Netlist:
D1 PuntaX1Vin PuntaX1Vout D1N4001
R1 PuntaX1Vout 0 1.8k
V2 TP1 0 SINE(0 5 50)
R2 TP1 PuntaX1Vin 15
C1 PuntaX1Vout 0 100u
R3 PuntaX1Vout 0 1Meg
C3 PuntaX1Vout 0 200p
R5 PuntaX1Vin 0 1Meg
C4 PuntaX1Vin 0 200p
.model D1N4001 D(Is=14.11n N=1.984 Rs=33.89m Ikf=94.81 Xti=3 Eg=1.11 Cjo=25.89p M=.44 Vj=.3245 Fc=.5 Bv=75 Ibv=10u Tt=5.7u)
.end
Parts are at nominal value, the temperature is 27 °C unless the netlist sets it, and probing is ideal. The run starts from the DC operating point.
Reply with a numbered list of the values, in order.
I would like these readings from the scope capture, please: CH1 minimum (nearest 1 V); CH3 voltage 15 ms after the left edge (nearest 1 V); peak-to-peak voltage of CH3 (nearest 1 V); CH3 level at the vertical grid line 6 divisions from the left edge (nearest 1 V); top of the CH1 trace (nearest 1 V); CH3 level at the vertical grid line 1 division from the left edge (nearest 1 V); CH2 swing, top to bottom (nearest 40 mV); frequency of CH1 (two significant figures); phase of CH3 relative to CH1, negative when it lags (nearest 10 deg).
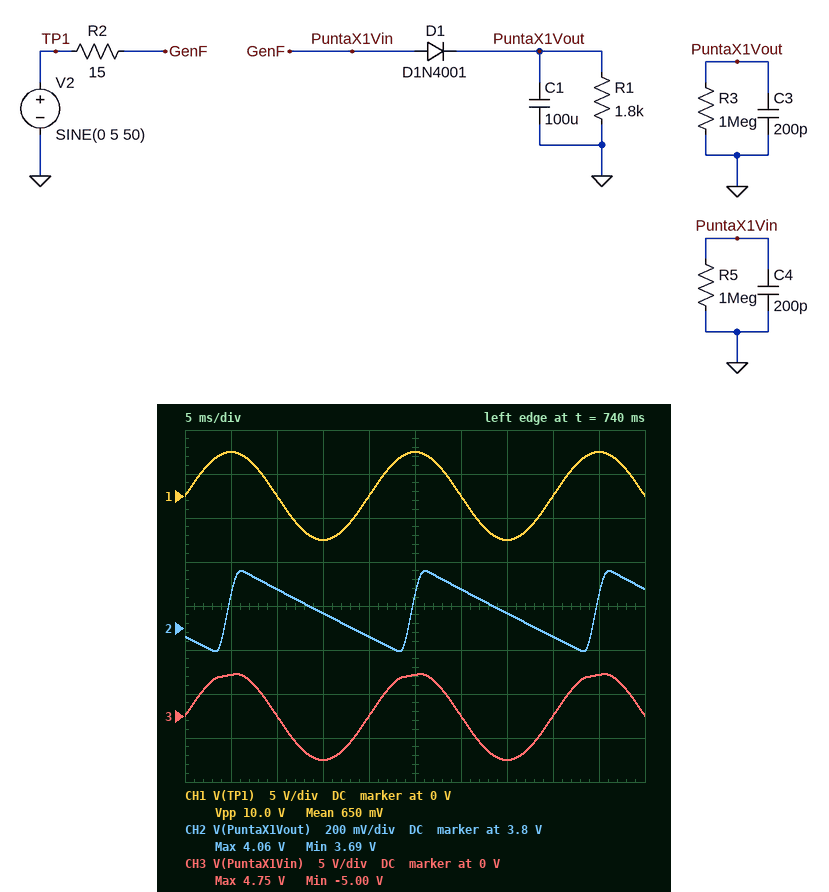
1. -5 V
2. -5 V
3. 10 V
4. 0 V
5. 5 V
6. 5 V
7. 360 mV
8. 50 Hz
9. 0 deg
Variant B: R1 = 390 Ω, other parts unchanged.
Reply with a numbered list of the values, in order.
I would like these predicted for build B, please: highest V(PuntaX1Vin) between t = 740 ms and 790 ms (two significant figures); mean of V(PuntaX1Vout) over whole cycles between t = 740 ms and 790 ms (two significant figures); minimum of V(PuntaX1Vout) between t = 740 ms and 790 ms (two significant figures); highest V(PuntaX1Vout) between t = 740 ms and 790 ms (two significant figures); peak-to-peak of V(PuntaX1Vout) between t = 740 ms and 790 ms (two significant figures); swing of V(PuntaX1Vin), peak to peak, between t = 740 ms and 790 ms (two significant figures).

1. 4.5 V
2. 3.1 V
3. 2.5 V
4. 3.8 V
5. 1.3 V
6. 9.5 V
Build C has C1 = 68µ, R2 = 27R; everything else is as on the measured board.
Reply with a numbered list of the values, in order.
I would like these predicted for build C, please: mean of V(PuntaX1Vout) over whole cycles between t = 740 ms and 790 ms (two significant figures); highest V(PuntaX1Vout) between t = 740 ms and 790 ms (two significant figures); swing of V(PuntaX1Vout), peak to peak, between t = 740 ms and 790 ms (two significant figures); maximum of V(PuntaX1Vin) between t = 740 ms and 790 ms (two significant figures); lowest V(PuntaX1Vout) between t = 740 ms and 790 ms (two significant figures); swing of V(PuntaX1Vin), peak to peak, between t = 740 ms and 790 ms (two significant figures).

1. 3.7 V
2. 4.0 V
3. 500 mV
4. 4.6 V
5. 3.5 V
6. 9.6 V
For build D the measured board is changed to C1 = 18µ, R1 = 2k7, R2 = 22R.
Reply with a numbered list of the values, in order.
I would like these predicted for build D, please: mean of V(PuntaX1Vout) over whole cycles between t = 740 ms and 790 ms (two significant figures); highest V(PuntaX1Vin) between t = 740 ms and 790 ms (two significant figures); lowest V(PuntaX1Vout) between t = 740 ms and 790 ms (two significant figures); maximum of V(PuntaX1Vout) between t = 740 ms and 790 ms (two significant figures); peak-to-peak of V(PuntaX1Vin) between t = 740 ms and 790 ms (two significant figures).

1. 3.6 V
2. 4.9 V
3. 3.0 V
4. 4.3 V
5. 9.9 V
